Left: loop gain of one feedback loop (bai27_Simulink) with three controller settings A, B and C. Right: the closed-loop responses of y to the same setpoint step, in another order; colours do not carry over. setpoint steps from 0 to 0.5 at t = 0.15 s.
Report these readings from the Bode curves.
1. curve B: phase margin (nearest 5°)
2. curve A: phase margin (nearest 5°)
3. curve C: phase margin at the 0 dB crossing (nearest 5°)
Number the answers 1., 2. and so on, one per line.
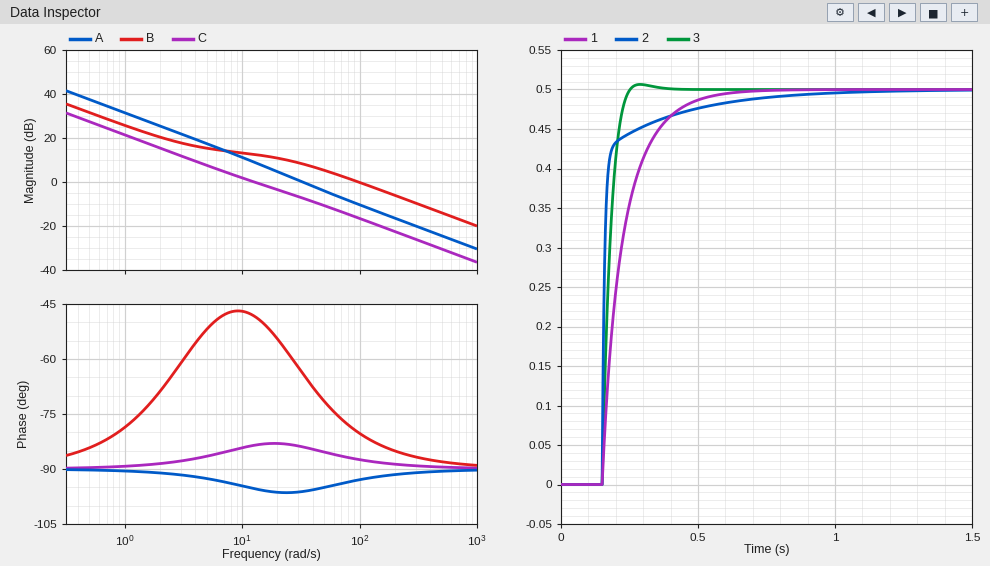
1. 100°
2. 85°
3. 95°
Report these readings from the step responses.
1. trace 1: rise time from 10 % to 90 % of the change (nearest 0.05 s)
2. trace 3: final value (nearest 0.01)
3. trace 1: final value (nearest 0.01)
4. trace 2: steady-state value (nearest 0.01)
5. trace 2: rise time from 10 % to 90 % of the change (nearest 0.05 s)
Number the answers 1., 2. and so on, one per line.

1. 0.20 s
2. 0.50
3. 0.50
4. 0.50
5. 0.15 s
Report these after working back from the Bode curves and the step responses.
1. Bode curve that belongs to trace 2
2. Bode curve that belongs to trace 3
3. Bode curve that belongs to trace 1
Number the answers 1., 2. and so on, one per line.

1. B
2. A
3. C
